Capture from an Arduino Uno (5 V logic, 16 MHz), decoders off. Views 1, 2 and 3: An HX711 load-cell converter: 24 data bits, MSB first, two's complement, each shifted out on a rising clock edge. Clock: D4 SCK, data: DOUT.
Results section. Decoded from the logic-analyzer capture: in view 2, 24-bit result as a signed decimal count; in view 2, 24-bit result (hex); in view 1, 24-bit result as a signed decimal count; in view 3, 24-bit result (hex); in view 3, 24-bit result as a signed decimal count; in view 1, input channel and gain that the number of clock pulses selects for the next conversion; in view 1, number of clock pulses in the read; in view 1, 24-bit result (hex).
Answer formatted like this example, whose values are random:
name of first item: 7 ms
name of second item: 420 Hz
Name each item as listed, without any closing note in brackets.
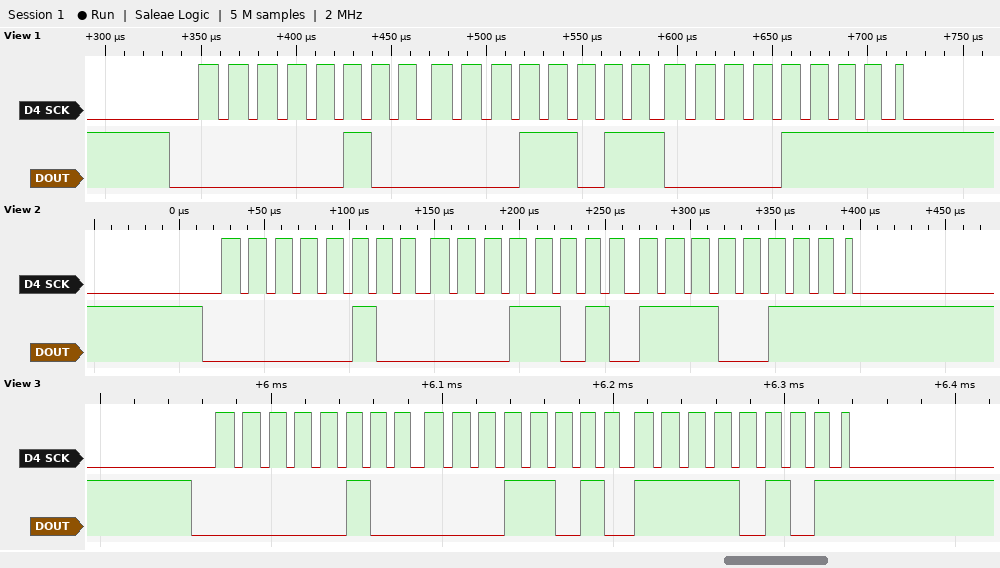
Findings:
in view 2, 24-bit result as a signed decimal count: 269031
in view 2, 24-bit result: 0x041AE7
in view 1, 24-bit result as a signed decimal count: 269071
in view 3, 24-bit result: 0x041AF5
in view 3, 24-bit result as a signed decimal count: 269045
in view 1, input channel and gain that the number of clock pulses selects for the next conversion: channel A, gain 128
in view 1, number of clock pulses in the read: 25
in view 1, 24-bit result: 0x041B0F
